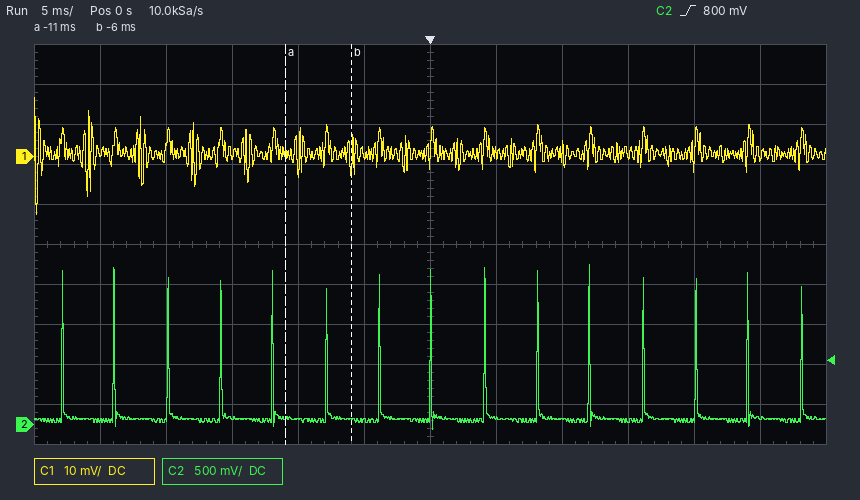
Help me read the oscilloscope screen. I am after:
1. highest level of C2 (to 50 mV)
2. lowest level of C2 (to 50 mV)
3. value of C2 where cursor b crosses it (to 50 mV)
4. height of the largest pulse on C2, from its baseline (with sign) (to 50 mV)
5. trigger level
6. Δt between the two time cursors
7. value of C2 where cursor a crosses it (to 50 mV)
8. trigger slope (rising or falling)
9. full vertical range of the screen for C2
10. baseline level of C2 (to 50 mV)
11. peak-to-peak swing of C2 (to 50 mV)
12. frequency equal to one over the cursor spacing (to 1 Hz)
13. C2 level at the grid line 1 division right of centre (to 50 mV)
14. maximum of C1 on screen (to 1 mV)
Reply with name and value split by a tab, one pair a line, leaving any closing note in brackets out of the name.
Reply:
highest level of C2	2.00 V
lowest level of C2	-50 mV
value of C2 where cursor b crosses it	50 mV
height of the largest pulse on C2, from its baseline (with sign)	+1.95 V
trigger level	800 mV
Δt between the two time cursors	5.0 ms
value of C2 where cursor a crosses it	100 mV
trigger slope	rising
full vertical range of the screen for C2	5 V
baseline level of C2	50 mV
peak-to-peak swing of C2	2.05 V
frequency equal to one over the cursor spacing	200 Hz
C2 level at the grid line 1 division right of centre	100 mV
maximum of C1 on screen	15 mV
